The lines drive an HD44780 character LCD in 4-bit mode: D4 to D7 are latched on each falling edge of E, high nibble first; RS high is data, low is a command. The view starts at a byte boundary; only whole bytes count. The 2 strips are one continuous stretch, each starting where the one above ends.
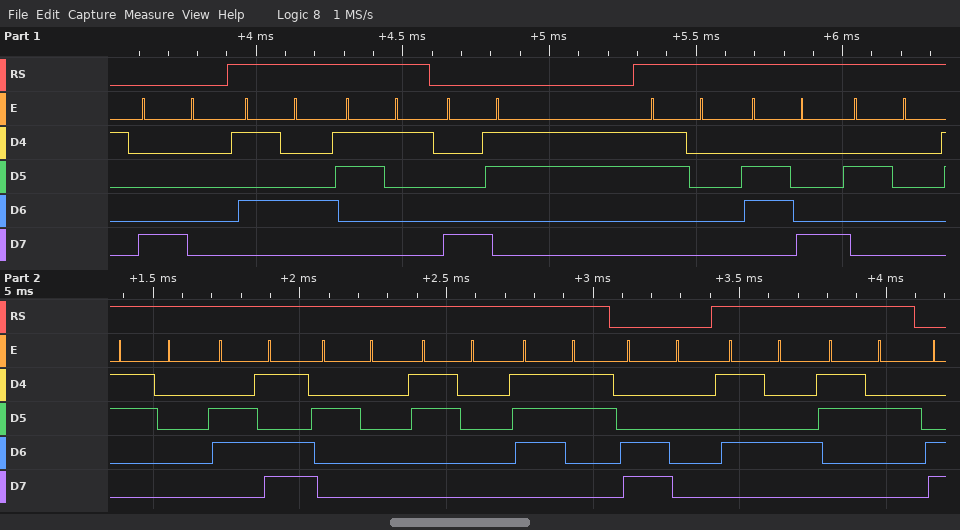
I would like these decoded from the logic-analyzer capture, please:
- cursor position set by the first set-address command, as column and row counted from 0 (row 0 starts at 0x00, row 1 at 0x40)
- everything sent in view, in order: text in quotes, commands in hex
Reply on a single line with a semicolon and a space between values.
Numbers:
column 0, row 0; 0x80 "T1" 0x83 "0h 0m 0s" 0xC0 "T2"
